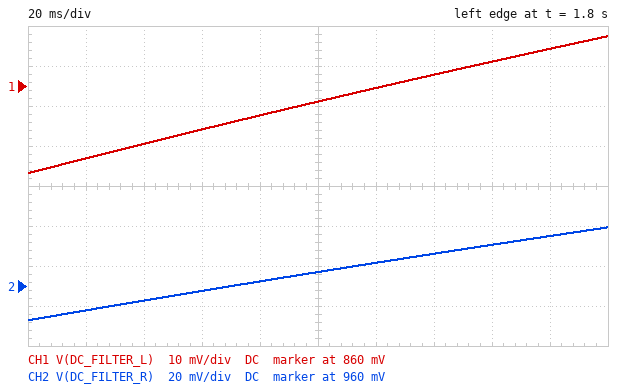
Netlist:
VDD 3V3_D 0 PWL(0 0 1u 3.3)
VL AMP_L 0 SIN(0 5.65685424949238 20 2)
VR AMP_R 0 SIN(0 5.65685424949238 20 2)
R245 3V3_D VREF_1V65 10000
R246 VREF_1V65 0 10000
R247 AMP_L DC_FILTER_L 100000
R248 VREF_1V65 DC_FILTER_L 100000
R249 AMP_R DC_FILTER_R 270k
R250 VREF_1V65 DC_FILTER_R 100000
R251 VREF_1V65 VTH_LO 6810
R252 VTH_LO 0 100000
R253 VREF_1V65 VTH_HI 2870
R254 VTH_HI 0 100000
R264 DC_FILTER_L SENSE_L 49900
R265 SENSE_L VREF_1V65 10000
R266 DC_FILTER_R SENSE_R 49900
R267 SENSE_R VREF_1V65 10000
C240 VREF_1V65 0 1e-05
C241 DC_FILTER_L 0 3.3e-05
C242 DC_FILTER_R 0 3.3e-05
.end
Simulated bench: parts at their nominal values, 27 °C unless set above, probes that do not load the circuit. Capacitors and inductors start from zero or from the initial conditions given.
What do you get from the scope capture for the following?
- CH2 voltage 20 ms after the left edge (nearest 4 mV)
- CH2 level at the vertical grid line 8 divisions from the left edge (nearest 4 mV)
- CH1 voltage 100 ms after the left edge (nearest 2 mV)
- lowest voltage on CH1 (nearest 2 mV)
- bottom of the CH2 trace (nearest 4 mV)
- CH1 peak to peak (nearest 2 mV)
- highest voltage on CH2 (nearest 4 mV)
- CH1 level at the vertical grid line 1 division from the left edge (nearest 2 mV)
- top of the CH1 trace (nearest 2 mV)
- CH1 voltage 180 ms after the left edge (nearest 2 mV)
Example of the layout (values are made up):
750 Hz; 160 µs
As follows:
948 mV; 980 mV; 856 mV; 838 mV; 944 mV; 34 mV; 988 mV; 842 mV; 872 mV; 870 mV
